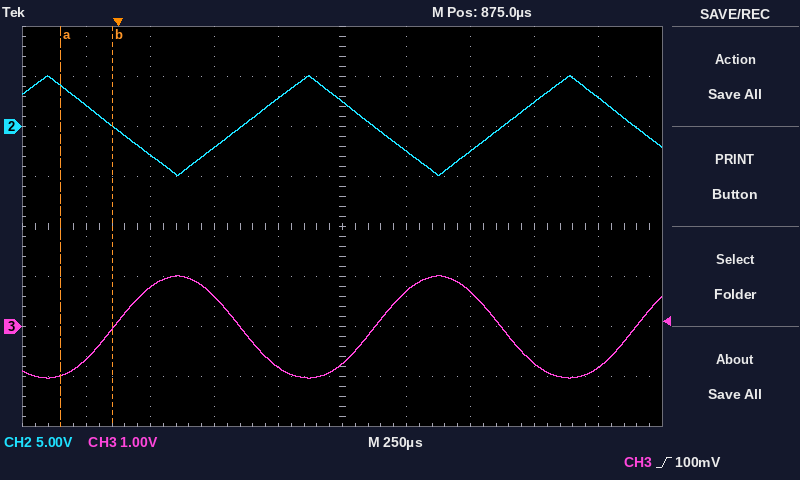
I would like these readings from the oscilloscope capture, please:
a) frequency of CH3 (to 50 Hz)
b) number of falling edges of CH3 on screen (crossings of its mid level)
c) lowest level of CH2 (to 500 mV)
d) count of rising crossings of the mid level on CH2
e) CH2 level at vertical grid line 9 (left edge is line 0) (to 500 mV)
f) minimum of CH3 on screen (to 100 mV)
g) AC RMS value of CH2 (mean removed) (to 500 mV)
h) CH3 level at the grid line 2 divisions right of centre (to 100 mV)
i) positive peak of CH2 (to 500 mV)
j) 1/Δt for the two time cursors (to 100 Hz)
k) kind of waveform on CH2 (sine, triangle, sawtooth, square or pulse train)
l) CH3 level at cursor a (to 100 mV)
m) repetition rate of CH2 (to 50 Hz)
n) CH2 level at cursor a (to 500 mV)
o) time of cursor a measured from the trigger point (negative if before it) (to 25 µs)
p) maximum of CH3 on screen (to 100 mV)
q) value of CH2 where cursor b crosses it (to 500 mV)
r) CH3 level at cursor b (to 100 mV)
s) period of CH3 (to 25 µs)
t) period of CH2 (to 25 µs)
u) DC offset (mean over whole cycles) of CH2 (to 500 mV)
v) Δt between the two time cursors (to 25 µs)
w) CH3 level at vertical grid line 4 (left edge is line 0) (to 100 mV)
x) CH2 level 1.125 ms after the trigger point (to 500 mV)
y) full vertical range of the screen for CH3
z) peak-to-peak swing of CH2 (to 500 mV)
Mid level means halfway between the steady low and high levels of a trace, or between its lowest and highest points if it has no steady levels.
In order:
1.00 kHz
2
-5.0 V
2
3.0 V
-1.0 V
3.0 V
700 mV
5.0 V
5.0 kHz
triangle
-1.0 V
1.00 kHz
4.0 V
-225 µs
1.0 V
0.0 V
0.0 V
1.025 ms
1.025 ms
0.0 V
200 µs
-800 mV
-2.5 V
8 V
10.0 V
